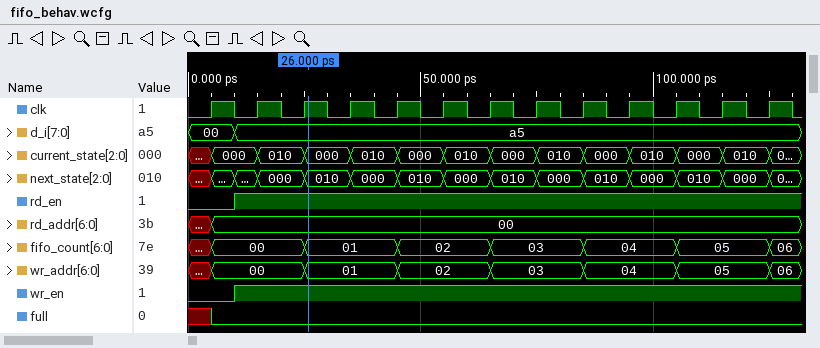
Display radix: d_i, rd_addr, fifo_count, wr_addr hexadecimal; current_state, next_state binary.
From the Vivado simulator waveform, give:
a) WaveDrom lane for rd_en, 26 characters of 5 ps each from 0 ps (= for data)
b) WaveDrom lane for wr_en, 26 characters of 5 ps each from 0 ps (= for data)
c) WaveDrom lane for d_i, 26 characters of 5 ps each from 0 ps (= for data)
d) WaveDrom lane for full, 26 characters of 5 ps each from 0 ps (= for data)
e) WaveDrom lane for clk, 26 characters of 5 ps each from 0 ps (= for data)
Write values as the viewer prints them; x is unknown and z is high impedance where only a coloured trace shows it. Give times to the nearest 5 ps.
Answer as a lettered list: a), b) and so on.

a) {name: 'rd_en', wave: '0.1.......................'}
b) {name: 'wr_en', wave: '0.1.......................'}
c) {name: 'd_i', wave: '=.=.......................', data: '00 a5'}
d) {name: 'full', wave: 'x0........................'}
e) {name: 'clk', wave: '01010101010101010101010101'}
